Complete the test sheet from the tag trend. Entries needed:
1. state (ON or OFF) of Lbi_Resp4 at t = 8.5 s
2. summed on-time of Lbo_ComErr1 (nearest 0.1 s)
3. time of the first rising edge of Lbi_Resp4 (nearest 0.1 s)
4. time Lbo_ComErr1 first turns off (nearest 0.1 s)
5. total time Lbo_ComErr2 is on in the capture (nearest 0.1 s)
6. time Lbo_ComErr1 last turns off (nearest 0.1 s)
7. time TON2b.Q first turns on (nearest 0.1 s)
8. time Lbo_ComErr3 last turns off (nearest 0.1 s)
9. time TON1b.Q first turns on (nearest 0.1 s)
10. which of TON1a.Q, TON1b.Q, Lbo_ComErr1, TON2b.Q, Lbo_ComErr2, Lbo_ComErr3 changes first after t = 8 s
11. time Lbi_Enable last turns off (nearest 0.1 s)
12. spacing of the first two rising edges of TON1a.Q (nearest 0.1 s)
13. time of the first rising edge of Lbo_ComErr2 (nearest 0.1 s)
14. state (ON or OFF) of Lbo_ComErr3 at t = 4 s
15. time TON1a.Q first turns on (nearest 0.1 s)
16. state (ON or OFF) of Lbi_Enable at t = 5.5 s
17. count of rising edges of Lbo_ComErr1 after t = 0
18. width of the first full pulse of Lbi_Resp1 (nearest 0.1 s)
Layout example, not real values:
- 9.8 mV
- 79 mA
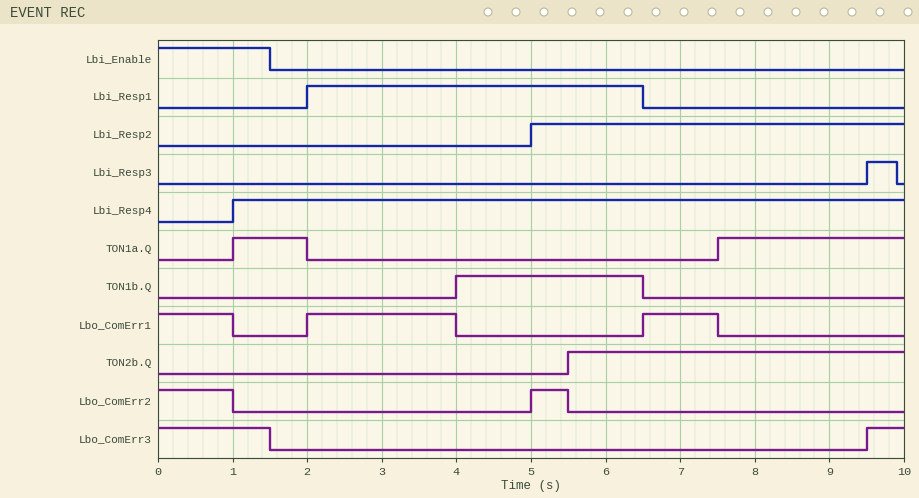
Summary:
- ON
- 4.0 s
- 1.0 s
- 1.0 s
- 1.5 s
- 7.5 s
- 5.5 s
- 1.5 s
- 4.0 s
- Lbo_ComErr3
- 1.5 s
- 6.5 s
- 5.0 s
- OFF
- 1.0 s
- OFF
- 2
- 4.5 s
